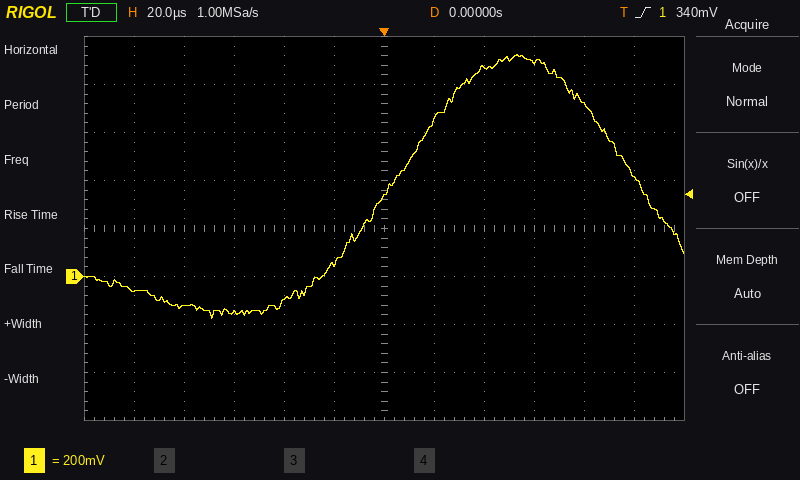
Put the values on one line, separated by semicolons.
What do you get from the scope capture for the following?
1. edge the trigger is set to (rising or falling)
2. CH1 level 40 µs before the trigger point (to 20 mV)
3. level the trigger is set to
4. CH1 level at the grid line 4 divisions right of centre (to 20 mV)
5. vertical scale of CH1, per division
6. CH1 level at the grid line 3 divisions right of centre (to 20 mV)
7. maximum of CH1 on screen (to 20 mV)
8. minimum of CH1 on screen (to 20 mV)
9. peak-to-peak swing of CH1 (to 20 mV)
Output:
rising; -100 mV; 340 mV; 720 mV; 200 mV; 900 mV; 920 mV; -180 mV; 1.10 V
